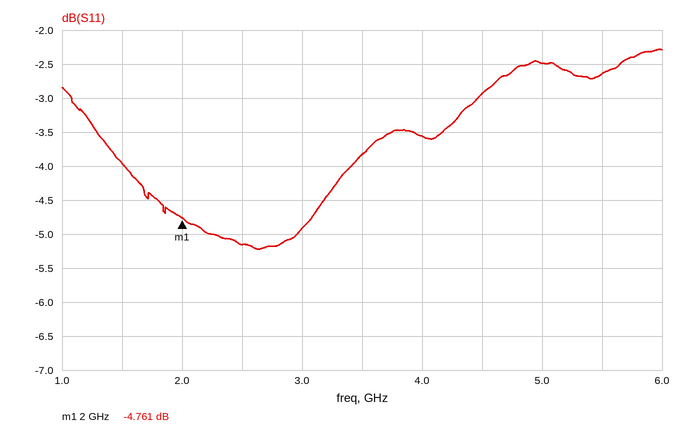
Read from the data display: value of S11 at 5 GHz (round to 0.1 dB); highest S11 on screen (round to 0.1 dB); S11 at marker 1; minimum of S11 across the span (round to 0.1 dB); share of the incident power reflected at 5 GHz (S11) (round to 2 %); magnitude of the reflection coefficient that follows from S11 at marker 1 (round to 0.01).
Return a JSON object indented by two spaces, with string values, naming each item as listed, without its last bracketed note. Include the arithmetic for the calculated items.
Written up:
{
  "value of S11 at 5 GHz": "-2.5 dB",
  "highest S11 on screen": "-2.3 dB",
  "S11 at marker 1": "-4.761 dB",
  "minimum of S11 across the span": "-5.2 dB",
  "share of the incident power reflected at 5 GHz (S11)": "10^(-2.5/10) ≈ 56 %",
  "magnitude of the reflection coefficient that follows from S11 at marker 1": "10^(-4.761/20) ≈ 0.58"
}
